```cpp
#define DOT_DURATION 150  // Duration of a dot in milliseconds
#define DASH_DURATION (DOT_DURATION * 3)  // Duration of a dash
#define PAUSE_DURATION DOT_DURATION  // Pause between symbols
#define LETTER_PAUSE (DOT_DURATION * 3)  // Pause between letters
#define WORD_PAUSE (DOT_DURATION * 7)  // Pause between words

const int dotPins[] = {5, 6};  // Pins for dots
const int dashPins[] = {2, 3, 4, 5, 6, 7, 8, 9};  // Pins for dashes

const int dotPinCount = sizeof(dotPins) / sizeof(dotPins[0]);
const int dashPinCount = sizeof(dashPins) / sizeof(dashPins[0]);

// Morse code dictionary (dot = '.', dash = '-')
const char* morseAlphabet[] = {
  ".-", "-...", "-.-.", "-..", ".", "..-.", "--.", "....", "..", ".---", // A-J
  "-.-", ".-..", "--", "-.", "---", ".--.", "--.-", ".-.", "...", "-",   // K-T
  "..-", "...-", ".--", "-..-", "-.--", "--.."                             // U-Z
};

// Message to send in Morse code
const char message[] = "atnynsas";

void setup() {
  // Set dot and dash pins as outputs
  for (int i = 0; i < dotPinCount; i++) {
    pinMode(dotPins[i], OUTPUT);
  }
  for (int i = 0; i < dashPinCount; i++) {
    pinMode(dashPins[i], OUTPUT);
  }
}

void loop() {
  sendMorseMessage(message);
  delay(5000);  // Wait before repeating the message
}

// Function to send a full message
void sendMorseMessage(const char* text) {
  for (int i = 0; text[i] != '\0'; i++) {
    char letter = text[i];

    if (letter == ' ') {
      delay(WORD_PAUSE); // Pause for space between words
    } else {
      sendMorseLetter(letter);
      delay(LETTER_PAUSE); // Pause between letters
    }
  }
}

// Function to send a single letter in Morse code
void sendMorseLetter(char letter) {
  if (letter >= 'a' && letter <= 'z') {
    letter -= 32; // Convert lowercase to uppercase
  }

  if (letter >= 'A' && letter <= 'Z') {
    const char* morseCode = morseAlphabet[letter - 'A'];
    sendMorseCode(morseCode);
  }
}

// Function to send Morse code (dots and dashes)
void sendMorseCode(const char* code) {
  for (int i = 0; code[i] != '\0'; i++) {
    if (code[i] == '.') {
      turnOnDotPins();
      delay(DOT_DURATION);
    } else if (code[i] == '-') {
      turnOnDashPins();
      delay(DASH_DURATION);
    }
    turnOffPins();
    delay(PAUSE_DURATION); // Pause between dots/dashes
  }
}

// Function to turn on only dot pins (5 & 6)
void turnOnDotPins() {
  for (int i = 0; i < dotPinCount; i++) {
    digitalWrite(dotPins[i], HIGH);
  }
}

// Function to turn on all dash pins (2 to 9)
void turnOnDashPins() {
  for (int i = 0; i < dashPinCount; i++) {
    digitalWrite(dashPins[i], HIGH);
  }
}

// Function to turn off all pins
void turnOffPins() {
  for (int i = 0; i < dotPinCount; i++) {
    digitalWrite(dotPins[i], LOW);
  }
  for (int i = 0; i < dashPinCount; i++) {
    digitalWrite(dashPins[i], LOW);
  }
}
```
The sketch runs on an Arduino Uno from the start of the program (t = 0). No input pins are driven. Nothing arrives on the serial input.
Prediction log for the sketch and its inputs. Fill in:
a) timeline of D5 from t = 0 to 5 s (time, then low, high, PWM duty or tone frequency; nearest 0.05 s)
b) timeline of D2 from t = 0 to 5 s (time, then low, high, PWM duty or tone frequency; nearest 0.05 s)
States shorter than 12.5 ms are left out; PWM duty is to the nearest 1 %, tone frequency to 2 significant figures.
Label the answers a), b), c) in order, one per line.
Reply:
a) 0 s high; 0.15 s low; 0.3 s high; 0.75 s low; 1.35 s high; 1.8 s low; 2.4 s high; 2.85 s low; 3 s high; 3.15 s low; 3.75 s high; 4.2 s low; 4.35 s high; 4.5 s low; 4.65 s high
b) 0 s low; 0.3 s high; 0.75 s low; 1.35 s high; 1.8 s low; 2.4 s high; 2.85 s low; 3.75 s high; 4.2 s low; 4.65 s high
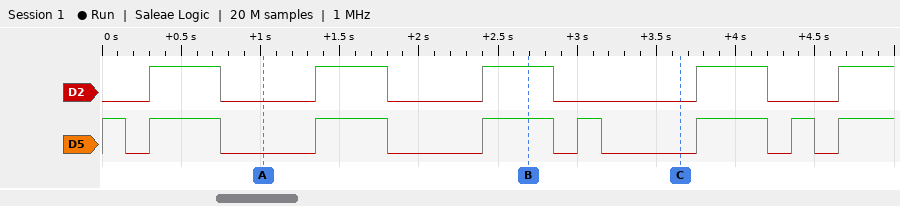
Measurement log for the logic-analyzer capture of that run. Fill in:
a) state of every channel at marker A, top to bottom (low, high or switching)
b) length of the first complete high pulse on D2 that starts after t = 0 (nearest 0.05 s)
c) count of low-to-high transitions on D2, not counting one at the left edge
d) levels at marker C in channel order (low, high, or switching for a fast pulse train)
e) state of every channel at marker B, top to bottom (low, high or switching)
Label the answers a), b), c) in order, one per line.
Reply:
a) D2 low, D5 low
b) 0.45 s
c) 5
d) D2 low, D5 low
e) D2 high, D5 high
